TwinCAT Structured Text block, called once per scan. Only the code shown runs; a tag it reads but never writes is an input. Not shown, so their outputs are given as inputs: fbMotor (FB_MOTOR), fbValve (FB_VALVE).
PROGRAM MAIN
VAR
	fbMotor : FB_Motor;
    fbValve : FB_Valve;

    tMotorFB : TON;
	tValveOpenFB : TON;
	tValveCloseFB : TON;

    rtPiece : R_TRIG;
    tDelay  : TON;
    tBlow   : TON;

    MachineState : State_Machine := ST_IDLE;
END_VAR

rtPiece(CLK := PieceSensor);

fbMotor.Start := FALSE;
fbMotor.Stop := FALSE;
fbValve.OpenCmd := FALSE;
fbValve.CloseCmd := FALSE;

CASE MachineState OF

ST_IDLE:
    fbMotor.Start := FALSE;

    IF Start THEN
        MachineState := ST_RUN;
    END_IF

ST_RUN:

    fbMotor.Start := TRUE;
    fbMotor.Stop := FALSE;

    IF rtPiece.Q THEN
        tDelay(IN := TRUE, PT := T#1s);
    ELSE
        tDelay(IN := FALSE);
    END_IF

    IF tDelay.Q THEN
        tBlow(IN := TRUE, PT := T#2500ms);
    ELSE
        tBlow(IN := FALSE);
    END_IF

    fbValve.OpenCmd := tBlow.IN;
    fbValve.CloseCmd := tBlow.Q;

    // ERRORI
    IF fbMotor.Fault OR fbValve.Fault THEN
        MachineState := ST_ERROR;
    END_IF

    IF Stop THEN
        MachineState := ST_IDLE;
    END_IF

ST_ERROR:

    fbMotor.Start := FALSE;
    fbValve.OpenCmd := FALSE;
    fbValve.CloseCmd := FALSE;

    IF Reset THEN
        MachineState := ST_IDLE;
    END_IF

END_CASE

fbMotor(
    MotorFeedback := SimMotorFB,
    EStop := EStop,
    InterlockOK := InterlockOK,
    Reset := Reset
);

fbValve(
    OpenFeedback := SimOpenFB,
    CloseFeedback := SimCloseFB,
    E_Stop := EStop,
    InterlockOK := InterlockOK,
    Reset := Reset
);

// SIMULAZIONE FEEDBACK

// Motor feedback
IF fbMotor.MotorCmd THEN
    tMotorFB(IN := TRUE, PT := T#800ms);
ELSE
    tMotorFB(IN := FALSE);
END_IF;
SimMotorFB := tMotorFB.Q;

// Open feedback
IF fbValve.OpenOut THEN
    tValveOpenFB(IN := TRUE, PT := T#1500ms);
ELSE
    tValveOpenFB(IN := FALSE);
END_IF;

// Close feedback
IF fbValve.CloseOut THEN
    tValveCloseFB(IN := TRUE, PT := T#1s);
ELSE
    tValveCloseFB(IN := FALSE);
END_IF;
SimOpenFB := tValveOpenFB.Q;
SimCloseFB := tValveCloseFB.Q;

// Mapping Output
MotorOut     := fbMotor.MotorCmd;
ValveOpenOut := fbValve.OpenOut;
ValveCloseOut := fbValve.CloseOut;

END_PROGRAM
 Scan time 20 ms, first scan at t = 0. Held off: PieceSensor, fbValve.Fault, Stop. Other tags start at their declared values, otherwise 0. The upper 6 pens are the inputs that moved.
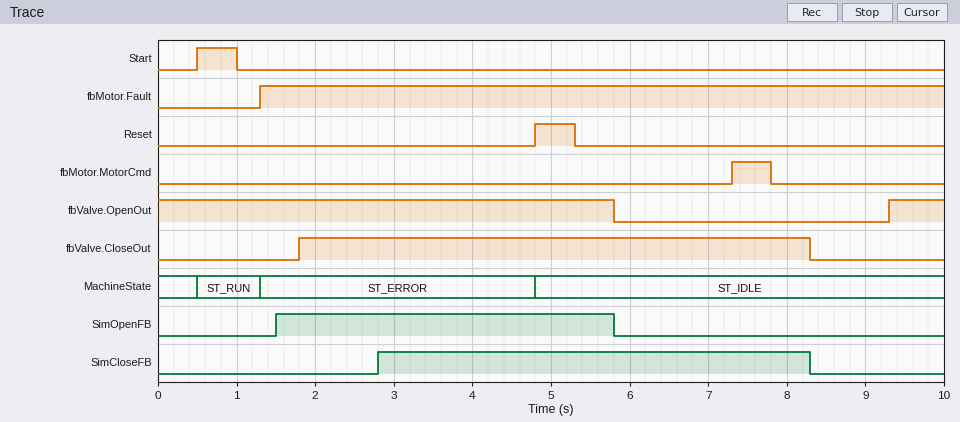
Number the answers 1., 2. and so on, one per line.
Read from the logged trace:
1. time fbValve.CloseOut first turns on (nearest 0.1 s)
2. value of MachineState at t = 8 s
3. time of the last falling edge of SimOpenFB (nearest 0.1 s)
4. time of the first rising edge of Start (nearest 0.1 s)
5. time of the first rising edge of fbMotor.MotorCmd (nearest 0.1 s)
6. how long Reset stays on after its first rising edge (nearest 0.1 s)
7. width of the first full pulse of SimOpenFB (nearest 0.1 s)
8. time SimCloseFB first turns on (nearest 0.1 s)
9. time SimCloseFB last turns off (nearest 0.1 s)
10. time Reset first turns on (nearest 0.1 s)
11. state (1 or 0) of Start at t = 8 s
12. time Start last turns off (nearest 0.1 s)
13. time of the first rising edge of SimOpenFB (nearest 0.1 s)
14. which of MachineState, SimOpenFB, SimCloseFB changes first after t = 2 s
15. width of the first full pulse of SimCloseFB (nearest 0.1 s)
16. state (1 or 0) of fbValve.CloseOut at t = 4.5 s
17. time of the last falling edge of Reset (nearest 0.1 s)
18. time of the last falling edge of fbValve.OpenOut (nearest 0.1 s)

1. 1.8 s
2. ST_IDLE
3. 5.8 s
4. 0.5 s
5. 7.3 s
6. 0.5 s
7. 4.3 s
8. 2.8 s
9. 8.3 s
10. 4.8 s
11. 0
12. 1.0 s
13. 1.5 s
14. SimCloseFB
15. 5.5 s
16. 1
17. 5.3 s
18. 5.8 s
